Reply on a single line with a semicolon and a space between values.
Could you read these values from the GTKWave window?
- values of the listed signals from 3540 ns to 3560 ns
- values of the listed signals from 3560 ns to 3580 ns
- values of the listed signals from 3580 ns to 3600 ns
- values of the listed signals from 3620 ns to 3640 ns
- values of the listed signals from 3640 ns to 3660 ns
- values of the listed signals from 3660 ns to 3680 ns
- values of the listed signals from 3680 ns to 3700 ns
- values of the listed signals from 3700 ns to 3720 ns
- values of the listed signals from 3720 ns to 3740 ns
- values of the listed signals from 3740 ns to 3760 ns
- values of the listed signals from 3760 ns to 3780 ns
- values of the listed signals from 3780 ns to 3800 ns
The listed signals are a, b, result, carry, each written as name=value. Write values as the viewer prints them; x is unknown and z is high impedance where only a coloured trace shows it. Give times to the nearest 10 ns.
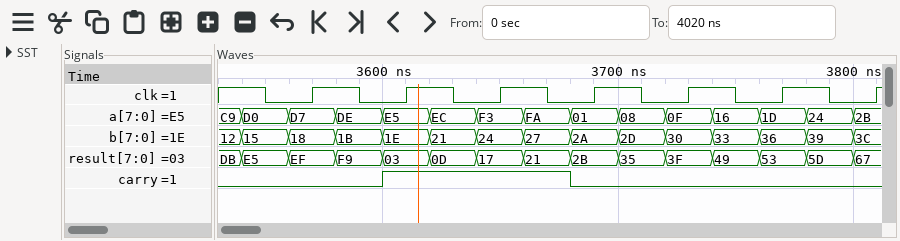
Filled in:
a=D0, b=15, result=E5, carry=0; a=D7, b=18, result=EF, carry=0; a=DE, b=1B, result=F9, carry=0; a=EC, b=21, result=0D, carry=1; a=F3, b=24, result=17, carry=1; a=FA, b=27, result=21, carry=1; a=01, b=2A, result=2B, carry=0; a=08, b=2D, result=35, carry=0; a=0F, b=30, result=3F, carry=0; a=16, b=33, result=49, carry=0; a=1D, b=36, result=53, carry=0; a=24, b=39, result=5D, carry=0
